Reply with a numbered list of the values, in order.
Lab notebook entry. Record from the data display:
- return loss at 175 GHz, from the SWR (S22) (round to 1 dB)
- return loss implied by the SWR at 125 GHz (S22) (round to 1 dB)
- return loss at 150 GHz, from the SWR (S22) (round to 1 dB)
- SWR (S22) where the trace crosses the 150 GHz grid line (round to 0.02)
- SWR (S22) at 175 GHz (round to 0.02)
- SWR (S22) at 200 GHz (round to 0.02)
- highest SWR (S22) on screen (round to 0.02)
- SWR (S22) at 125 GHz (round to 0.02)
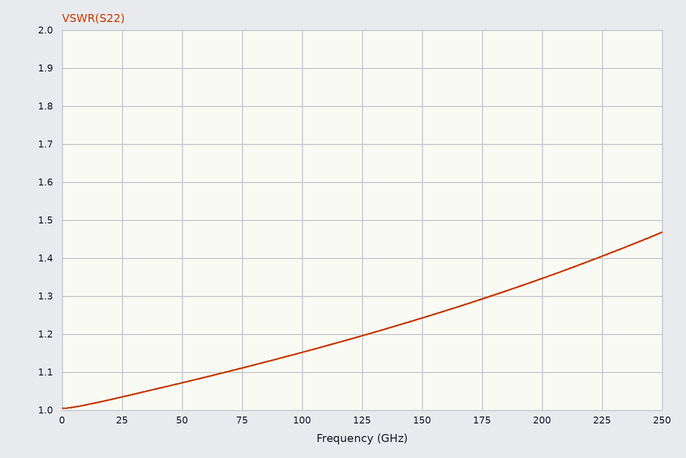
1. 18 dB
2. 21 dB
3. 19 dB
4. 1.24
5. 1.30
6. 1.34
7. 1.46
8. 1.20
